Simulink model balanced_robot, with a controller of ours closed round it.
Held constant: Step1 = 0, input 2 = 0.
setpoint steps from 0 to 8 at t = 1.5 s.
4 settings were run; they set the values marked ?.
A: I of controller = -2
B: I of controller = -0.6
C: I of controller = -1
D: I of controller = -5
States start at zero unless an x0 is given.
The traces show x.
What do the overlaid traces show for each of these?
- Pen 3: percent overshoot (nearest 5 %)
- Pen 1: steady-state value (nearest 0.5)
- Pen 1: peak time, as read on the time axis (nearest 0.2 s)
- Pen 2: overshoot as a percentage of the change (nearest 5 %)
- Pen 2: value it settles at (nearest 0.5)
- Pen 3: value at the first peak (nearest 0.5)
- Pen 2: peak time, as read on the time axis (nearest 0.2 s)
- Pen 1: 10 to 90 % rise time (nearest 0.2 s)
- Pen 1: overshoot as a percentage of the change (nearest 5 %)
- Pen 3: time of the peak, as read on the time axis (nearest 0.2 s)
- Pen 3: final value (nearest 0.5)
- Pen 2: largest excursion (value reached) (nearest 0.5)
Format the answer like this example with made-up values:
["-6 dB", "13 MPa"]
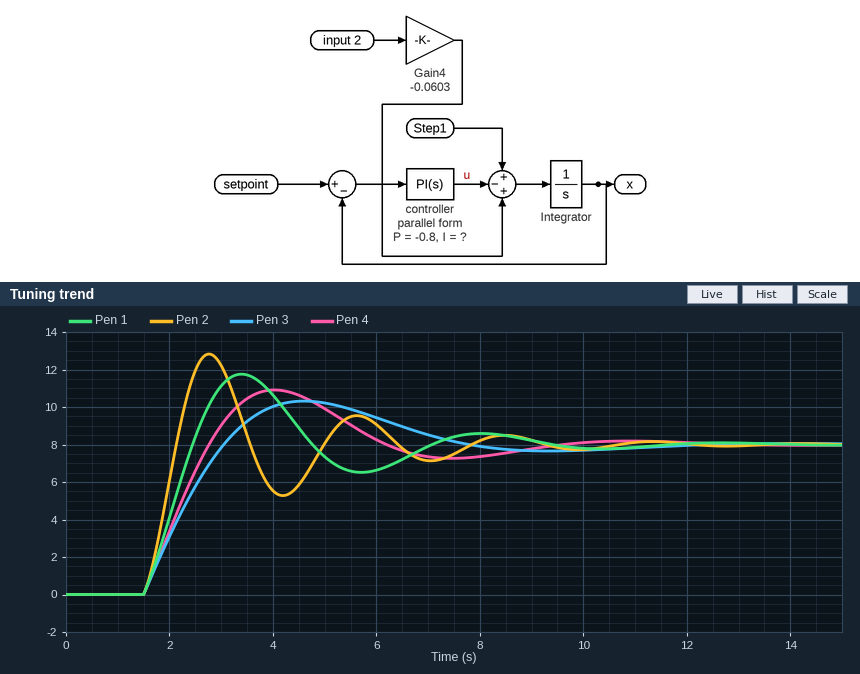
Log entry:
["30 %", "8.0", "3.4 s", "60 %", "8.0", "10.5", "2.8 s", "0.8 s", "45 %", "4.6 s", "8.0", "13.0"]
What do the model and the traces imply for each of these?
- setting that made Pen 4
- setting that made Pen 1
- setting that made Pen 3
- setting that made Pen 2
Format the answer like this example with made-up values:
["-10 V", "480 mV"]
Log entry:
["C", "A", "B", "D"]
